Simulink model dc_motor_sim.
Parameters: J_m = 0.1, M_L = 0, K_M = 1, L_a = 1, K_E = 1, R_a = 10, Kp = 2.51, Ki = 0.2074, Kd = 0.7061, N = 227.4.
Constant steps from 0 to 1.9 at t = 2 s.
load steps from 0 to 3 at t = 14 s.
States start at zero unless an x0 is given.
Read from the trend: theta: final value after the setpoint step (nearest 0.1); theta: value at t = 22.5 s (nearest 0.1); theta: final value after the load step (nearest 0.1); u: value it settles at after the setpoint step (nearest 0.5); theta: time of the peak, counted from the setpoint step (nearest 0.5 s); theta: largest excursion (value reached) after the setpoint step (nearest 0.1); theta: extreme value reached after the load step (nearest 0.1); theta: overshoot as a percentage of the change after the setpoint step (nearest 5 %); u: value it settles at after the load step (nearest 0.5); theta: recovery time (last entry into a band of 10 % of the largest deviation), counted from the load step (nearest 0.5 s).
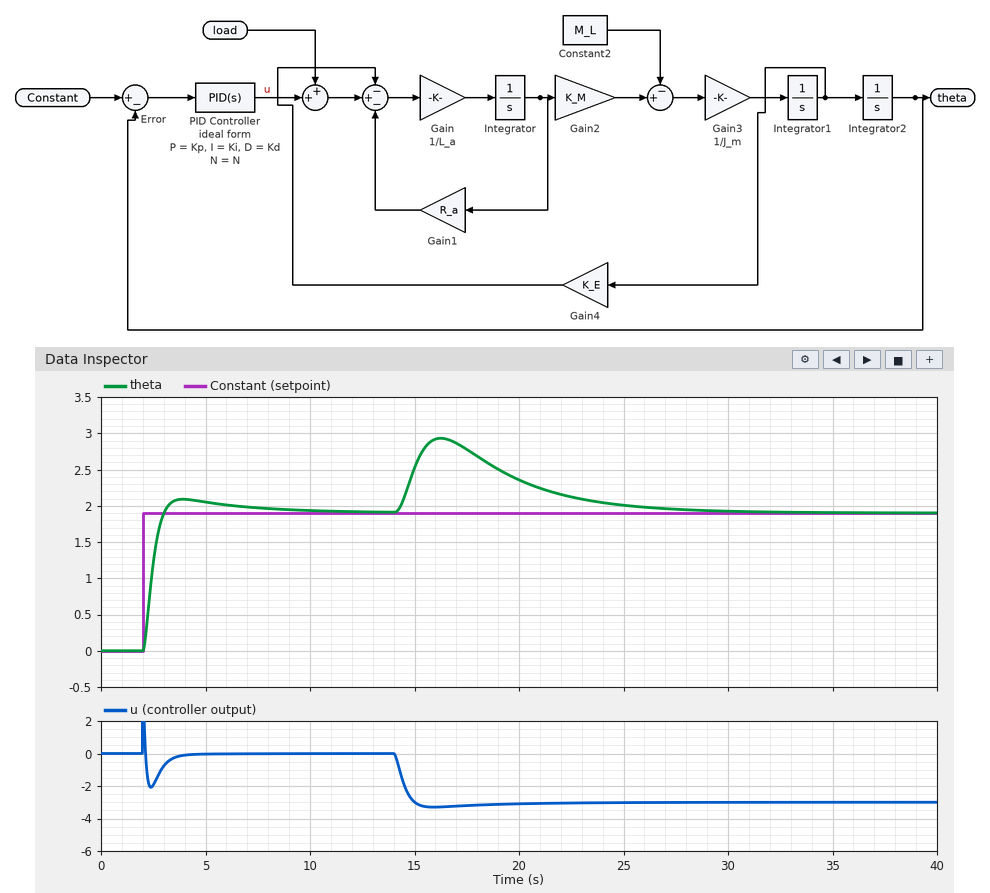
1.9
2.1
1.9
0.0
2.0 s
2.1
2.9
10 %
-3.0
11.0 s
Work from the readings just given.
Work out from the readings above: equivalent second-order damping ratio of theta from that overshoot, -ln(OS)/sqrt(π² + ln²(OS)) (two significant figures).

0.59
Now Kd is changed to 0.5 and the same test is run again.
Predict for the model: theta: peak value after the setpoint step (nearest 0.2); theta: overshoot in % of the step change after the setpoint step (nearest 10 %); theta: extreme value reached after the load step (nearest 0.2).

2.2
20 %
3.0
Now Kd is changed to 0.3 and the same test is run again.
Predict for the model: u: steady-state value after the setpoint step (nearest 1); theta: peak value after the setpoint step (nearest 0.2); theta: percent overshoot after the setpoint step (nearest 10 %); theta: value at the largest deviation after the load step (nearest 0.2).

0
2.4
30 %
3.2
